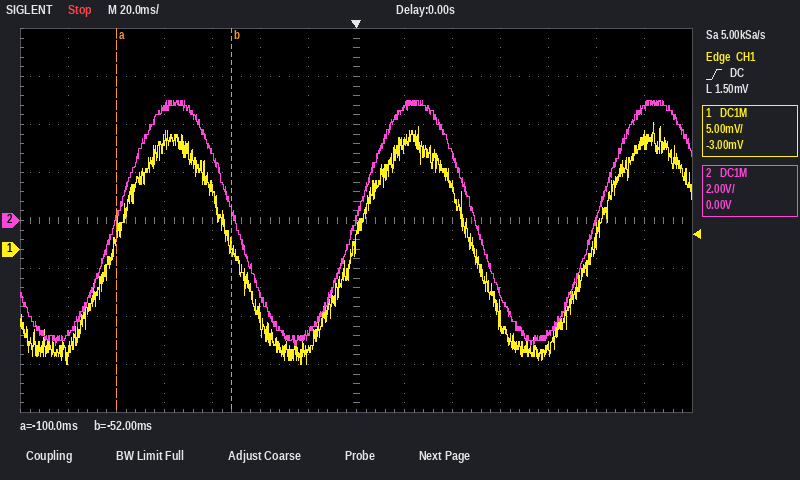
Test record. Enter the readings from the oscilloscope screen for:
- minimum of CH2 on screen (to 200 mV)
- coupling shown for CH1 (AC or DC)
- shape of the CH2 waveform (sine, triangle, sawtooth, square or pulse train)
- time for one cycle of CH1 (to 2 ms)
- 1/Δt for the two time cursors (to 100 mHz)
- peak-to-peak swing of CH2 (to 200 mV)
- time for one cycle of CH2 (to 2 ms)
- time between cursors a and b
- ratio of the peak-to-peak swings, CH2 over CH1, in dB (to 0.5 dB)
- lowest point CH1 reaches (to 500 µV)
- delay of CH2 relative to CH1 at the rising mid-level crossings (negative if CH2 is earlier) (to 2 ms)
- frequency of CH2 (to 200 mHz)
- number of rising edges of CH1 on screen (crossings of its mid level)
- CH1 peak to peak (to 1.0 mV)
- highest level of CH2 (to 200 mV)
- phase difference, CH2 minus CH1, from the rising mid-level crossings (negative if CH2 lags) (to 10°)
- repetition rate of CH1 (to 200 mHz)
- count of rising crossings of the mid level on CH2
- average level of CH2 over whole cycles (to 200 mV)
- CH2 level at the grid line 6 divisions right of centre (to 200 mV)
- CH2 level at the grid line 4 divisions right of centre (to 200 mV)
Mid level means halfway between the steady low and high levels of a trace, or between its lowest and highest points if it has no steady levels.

-5.2 V
DC
sine
100 ms
20.8 Hz
10.2 V
100 ms
48 ms
52.0 dB
-12.0 mV
0 ms
10.0 Hz
3
25.0 mV
5.0 V
0°
10.0 Hz
3
0.0 V
4.8 V
-4.8 V
